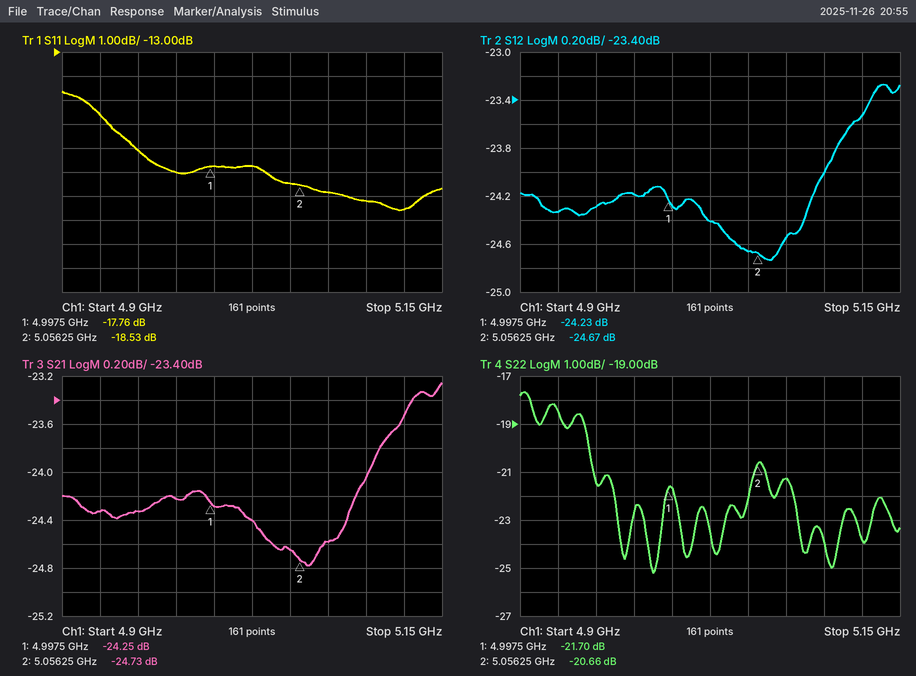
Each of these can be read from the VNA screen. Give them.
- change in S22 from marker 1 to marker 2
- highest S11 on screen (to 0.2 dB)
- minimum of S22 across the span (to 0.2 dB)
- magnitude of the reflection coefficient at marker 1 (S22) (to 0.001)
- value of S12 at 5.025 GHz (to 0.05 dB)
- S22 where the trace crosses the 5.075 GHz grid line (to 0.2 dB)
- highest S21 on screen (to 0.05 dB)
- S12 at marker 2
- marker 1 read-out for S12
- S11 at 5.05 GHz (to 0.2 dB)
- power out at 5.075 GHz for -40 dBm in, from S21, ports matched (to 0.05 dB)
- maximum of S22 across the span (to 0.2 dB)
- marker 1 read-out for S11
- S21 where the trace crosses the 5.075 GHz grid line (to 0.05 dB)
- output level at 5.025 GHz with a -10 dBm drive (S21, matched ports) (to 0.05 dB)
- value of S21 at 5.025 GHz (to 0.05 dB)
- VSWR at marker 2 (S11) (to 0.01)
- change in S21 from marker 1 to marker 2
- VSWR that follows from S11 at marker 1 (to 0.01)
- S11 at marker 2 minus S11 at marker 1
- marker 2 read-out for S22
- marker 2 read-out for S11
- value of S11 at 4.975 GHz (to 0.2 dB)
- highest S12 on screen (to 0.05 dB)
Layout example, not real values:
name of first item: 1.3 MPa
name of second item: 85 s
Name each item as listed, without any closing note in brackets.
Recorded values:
change in S22 from marker 1 to marker 2: 1.04 dB
highest S11 on screen: -14.6 dB
minimum of S22 across the span: -25.2 dB
magnitude of the reflection coefficient at marker 1 (S22): 0.082
value of S12 at 5.025 GHz: -24.40 dB
S22 where the trace crosses the 5.075 GHz grid line: -21.2 dB
highest S21 on screen: -23.25 dB
S12 at marker 2: -24.67 dB
marker 1 read-out for S12: -24.23 dB
S11 at 5.05 GHz: -18.4 dB
power out at 5.075 GHz for -40 dBm in, from S21, ports matched: -64.60 dBm
maximum of S22 across the span: -17.6 dB
marker 1 read-out for S11: -17.76 dB
S21 where the trace crosses the 5.075 GHz grid line: -24.60 dB
output level at 5.025 GHz with a -10 dBm drive (S21, matched ports): -34.40 dBm
value of S21 at 5.025 GHz: -24.40 dB
VSWR at marker 2 (S11): 1.27
change in S21 from marker 1 to marker 2: -0.48 dB
VSWR that follows from S11 at marker 1: 1.30
S11 at marker 2 minus S11 at marker 1: -0.77 dB
marker 2 read-out for S22: -20.66 dB
marker 2 read-out for S11: -18.53 dB
value of S11 at 4.975 GHz: -18.0 dB
highest S12 on screen: -23.25 dB
